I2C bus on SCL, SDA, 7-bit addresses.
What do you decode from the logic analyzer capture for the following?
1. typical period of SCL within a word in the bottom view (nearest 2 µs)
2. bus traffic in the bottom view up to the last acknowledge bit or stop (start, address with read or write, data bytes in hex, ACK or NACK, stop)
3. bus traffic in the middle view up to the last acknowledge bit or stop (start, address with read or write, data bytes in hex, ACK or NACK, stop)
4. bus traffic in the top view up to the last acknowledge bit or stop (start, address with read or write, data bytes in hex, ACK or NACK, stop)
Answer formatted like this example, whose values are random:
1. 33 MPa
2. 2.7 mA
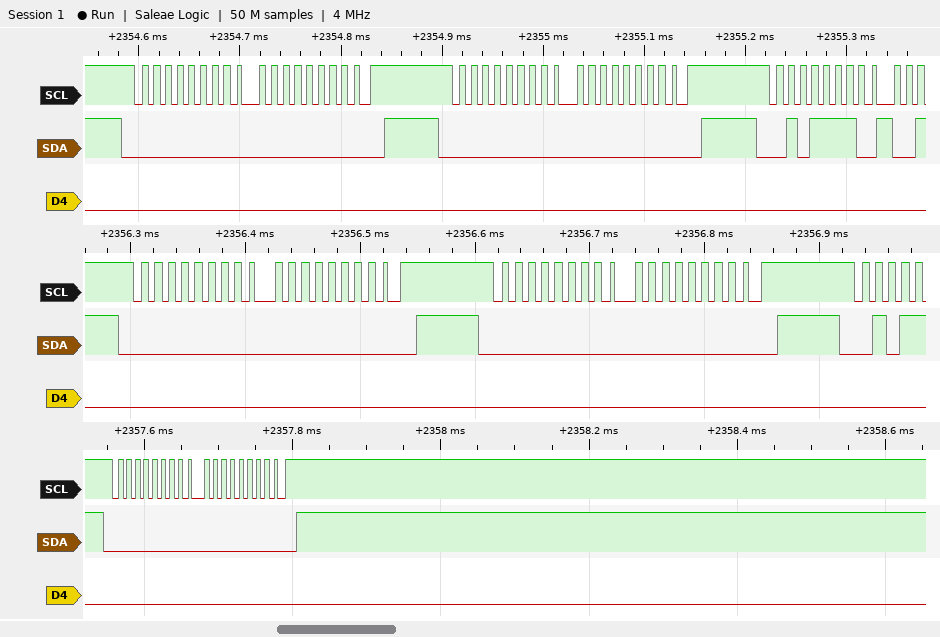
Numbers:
1. 12 µs
2. start, address 00 write ACK, 00 ACK, stop
3. start, address 00 write ACK, 00 ACK, stop, start, address 00 write ACK, 00 ACK, stop
4. start, address 00 write ACK, 00 ACK, stop, start, address 00 write ACK, 00 ACK, stop, start, address 2F write ACK
